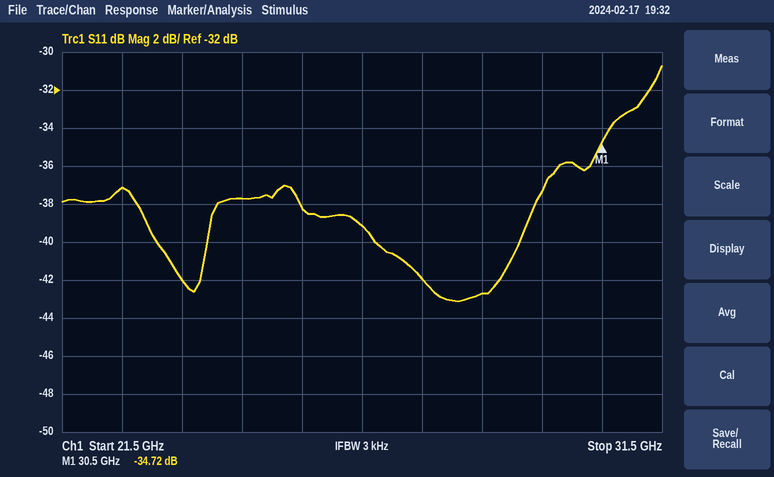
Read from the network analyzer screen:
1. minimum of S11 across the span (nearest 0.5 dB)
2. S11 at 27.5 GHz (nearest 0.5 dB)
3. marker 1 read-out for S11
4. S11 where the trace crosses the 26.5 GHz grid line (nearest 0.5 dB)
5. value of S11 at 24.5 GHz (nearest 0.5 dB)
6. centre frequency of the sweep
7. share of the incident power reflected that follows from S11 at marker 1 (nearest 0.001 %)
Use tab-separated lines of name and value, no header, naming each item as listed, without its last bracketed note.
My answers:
minimum of S11 across the span	-43.0 dB
S11 at 27.5 GHz	-42.0 dB
marker 1 read-out for S11	-34.72 dB
S11 where the trace crosses the 26.5 GHz grid line	-39.0 dB
value of S11 at 24.5 GHz	-37.5 dB
centre frequency of the sweep	26.5 GHz
share of the incident power reflected that follows from S11 at marker 1	0.034 %
